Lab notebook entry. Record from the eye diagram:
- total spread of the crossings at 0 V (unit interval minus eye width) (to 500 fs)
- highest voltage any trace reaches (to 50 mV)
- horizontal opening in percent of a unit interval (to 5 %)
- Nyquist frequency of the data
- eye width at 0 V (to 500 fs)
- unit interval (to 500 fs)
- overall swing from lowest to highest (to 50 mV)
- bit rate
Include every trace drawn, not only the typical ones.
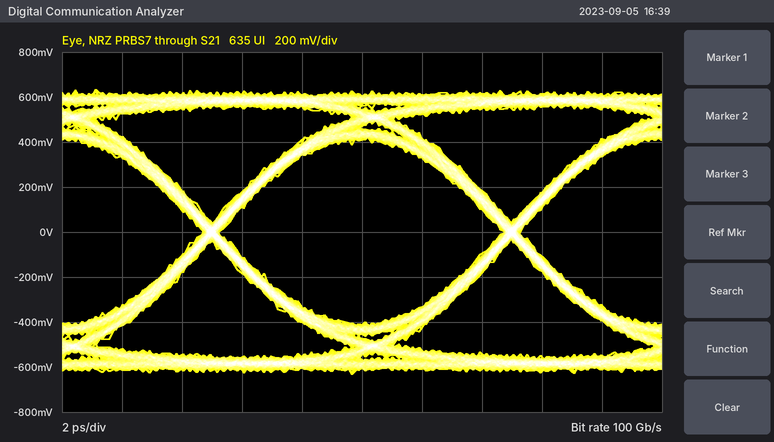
500 fs
650 mV
95 %
50 GHz
9.5 ps
10.0 ps
1.25 V
100 Gb/s
